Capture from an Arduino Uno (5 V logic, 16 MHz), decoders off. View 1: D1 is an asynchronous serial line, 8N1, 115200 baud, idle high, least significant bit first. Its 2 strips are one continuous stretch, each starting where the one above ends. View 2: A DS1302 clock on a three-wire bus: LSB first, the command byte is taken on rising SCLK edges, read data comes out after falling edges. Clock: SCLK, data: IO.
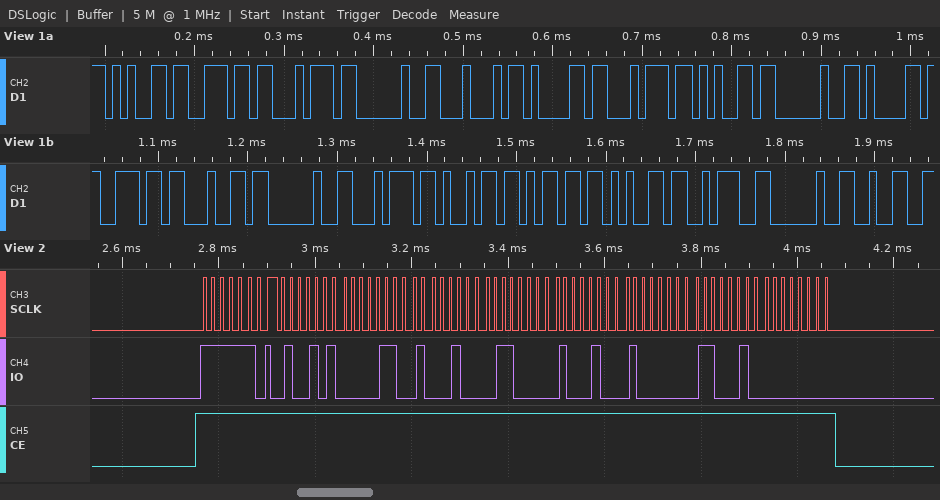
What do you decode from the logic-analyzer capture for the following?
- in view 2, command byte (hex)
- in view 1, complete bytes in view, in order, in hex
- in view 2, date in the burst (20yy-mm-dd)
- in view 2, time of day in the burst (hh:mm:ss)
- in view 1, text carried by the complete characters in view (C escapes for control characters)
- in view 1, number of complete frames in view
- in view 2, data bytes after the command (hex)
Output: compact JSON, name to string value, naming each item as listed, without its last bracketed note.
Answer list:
{"in view 2, command byte": "0xBF", "in view 1, complete bytes in view, in order, in hex": "0x65 0x6E 0x74 0x20 0x44 0x61 0x74 0x65 0x20 0x61 0x6E 0x64 0x20 0x74 0x69 0x6D 0x65 0x3A 0x20 0x32", "in view 2, date in the burst": "2023-11-06", "in view 2, time of day in the burst": "11:30:52", "in view 1, text carried by the complete characters in view": "\"ent Date and time: 2\"", "in view 1, number of complete frames in view": "20", "in view 2, data bytes after the command": "52 30 11 06 11 01 23 00"}
